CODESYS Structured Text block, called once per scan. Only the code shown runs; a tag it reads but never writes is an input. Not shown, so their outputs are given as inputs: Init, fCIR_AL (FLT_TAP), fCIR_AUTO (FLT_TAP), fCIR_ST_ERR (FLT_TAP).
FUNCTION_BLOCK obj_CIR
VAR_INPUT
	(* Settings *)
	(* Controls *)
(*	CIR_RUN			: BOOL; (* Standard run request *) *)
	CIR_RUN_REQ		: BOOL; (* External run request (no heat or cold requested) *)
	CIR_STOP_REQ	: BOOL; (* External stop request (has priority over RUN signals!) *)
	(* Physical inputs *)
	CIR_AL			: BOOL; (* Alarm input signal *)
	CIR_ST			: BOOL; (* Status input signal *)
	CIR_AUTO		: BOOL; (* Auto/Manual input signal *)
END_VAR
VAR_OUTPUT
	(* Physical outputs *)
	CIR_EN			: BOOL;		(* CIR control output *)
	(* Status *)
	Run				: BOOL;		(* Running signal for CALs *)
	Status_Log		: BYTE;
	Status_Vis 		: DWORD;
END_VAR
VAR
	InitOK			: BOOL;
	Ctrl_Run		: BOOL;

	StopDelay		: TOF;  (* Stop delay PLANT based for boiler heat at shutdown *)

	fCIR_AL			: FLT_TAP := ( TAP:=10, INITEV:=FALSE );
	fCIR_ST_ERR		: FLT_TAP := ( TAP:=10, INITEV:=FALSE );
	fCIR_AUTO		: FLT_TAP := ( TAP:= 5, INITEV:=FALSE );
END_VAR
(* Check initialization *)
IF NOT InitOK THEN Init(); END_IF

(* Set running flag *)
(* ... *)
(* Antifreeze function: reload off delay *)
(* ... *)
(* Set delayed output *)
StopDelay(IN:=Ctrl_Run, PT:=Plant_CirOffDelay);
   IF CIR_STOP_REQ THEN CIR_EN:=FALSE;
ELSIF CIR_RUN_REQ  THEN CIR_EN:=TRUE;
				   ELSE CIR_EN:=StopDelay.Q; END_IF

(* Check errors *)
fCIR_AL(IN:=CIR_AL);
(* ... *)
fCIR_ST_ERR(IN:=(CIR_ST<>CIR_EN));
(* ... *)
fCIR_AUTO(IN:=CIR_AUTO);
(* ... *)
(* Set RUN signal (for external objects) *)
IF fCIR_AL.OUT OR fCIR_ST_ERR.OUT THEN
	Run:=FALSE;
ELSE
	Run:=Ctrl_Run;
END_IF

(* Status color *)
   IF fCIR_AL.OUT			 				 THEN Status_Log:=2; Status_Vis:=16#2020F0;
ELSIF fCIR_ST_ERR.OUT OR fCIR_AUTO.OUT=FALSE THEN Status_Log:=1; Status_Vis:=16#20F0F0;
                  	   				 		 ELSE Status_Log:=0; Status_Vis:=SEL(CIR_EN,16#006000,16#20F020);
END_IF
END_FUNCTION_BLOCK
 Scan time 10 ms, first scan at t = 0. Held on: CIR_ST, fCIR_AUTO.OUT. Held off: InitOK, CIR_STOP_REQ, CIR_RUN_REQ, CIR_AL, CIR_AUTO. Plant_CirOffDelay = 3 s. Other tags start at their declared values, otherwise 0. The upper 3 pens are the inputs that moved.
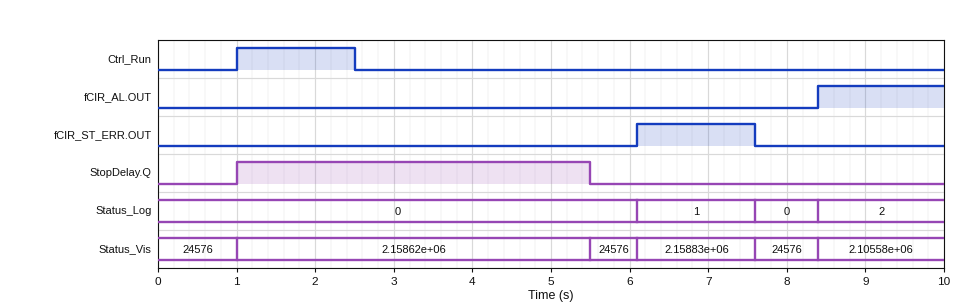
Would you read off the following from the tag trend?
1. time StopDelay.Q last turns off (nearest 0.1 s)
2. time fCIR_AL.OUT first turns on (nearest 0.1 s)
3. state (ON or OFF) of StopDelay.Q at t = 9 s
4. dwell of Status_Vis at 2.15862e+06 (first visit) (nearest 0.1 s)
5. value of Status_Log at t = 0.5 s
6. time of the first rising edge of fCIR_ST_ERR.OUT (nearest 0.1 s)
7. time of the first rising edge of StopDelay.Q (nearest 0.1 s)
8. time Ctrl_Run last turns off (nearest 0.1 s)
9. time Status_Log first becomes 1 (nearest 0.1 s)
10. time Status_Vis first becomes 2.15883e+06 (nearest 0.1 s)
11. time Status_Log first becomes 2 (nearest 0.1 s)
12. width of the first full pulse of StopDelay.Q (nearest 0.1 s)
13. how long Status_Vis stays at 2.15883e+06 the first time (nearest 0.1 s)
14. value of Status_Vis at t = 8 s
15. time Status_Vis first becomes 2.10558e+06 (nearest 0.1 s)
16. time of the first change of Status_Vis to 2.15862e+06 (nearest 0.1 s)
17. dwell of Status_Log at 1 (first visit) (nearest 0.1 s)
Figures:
5.5 s
8.4 s
OFF
4.5 s
0
6.1 s
1.0 s
2.5 s
6.1 s
6.1 s
8.4 s
4.5 s
1.5 s
24576
8.4 s
1.0 s
1.5 s
